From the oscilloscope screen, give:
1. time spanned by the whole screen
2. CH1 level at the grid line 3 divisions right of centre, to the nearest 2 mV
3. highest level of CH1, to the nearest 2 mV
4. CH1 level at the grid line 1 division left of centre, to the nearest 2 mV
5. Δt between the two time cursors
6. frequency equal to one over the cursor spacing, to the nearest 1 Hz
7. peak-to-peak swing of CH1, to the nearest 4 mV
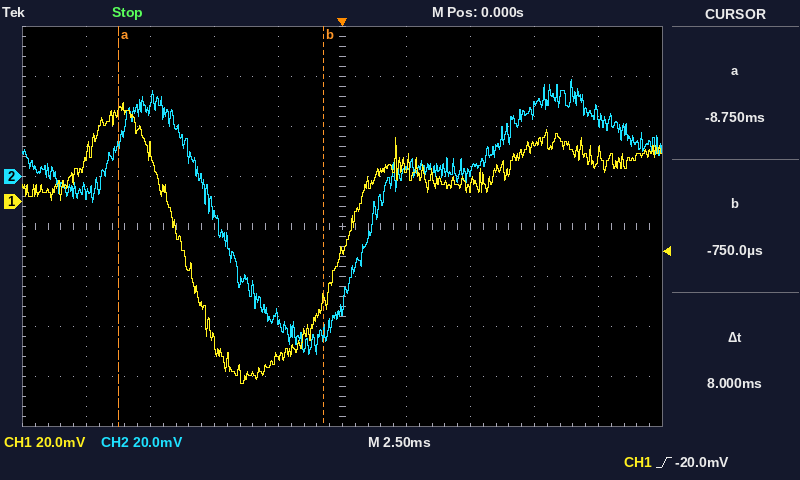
25 ms
22 mV
40 mV
-62 mV
8 ms
125 Hz
112 mV
